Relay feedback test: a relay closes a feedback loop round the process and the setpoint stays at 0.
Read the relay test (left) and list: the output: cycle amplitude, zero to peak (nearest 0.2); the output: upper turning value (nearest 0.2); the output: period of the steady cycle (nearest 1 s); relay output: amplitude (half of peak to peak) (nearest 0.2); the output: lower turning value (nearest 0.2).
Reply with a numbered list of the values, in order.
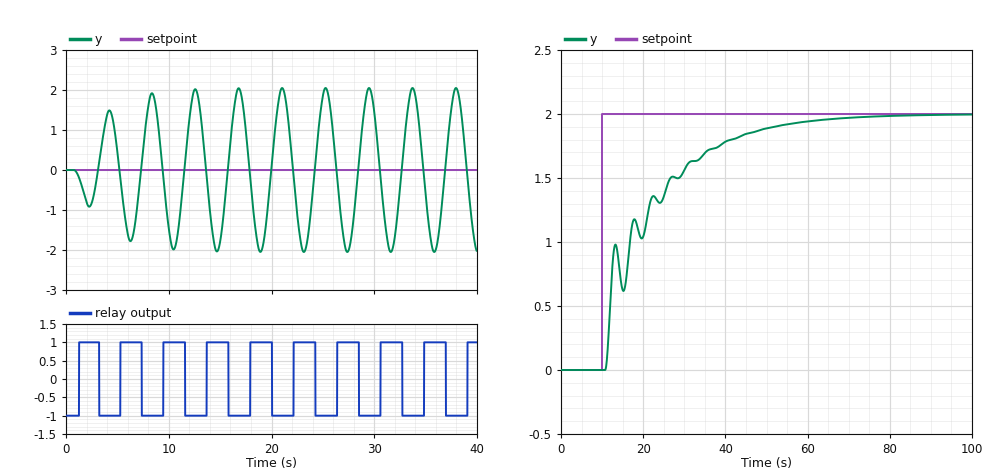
1. 2.0
2. 2.0
3. 4 s
4. 1.0
5. -2.0
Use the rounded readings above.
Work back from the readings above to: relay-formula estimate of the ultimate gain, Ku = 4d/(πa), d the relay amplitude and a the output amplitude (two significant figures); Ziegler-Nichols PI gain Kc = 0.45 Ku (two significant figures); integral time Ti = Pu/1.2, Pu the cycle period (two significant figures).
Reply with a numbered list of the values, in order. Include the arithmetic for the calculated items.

1. 4 × 1 / (π × 2) = 0.64
2. 0.45 × 0.64 = 0.29
3. 4 / 1.2 = 3.3 s
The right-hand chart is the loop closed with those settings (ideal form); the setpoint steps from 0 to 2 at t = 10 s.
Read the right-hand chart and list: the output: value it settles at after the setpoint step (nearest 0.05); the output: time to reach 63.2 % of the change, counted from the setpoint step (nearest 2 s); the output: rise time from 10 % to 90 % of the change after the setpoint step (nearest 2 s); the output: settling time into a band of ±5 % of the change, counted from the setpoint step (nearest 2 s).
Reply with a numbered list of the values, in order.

1. 2.00
2. 12 s
3. 30 s
4. 42 s
